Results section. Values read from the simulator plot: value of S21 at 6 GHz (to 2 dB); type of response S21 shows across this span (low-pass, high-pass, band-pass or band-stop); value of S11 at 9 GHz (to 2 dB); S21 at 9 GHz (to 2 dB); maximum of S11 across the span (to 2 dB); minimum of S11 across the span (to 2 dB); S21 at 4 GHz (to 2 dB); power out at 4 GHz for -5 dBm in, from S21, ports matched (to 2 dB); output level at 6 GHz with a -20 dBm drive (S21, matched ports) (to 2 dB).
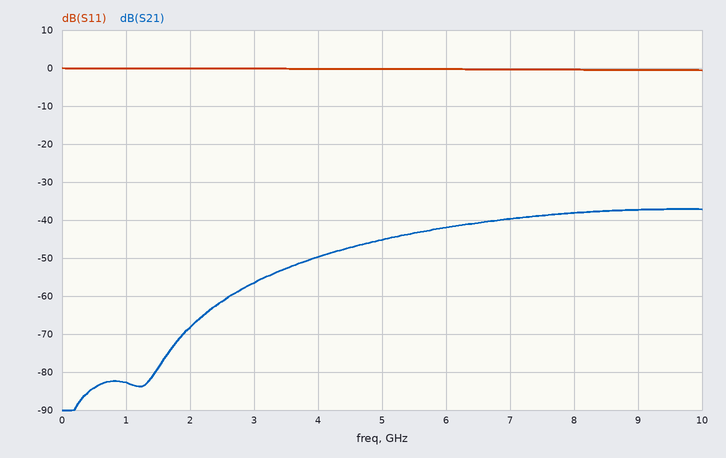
-42 dB
high-pass
0 dB
-38 dB
0 dB
0 dB
-50 dB
-54 dBm
-62 dBm
